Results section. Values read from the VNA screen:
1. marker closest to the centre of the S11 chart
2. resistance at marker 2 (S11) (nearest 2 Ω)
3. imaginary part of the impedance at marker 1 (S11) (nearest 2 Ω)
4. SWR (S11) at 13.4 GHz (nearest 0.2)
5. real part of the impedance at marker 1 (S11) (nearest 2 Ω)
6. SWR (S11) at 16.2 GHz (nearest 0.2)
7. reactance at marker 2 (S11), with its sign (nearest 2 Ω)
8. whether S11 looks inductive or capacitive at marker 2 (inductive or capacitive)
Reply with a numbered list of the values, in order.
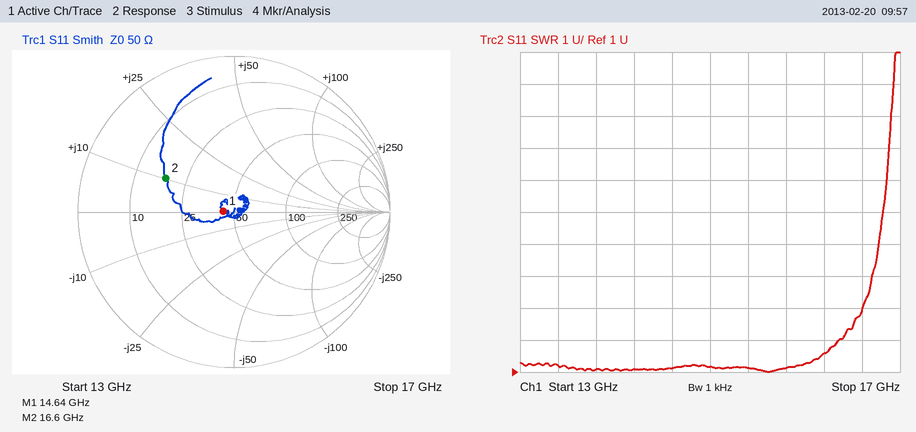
1. marker 1
2. 18 Ω
3. 0 Ω
4. 1.2
5. 44 Ω
6. 1.6
7. +10 Ω
8. inductive
